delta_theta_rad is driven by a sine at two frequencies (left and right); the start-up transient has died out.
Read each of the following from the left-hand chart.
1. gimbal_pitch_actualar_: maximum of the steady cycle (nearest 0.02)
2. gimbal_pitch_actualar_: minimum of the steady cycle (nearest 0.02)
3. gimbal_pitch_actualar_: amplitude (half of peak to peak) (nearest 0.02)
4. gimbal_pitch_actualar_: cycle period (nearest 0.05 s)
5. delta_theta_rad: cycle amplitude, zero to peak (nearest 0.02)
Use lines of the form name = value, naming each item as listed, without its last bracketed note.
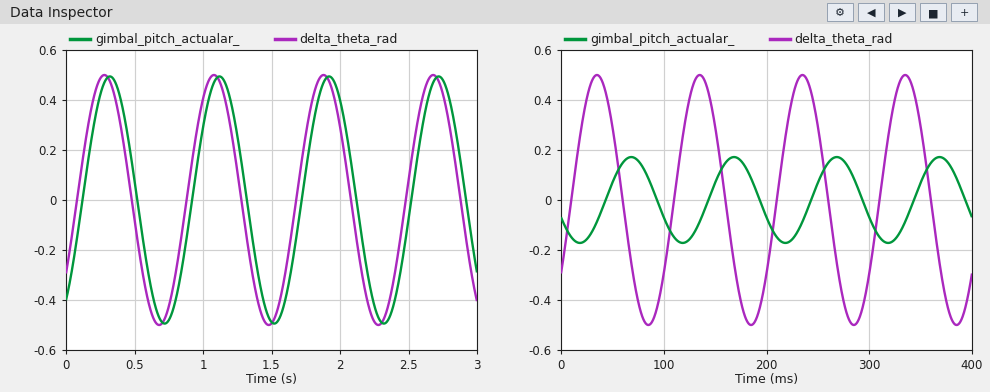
gimbal_pitch_actualar_: maximum of the steady cycle = 0.50
gimbal_pitch_actualar_: minimum of the steady cycle = -0.50
gimbal_pitch_actualar_: amplitude (half of peak to peak) = 0.50
gimbal_pitch_actualar_: cycle period = 0.80 s
delta_theta_rad: cycle amplitude, zero to peak = 0.50
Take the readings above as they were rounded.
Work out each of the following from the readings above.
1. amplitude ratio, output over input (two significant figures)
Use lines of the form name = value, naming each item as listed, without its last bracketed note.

amplitude ratio, output over input = 1.0
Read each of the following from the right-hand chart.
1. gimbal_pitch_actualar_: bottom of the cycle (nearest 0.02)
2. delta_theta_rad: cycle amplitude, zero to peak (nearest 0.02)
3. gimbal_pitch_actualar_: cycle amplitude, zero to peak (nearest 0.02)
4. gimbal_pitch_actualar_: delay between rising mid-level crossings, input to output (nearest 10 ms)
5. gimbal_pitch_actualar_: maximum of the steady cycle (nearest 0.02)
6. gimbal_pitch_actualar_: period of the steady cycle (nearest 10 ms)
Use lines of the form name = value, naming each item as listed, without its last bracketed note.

gimbal_pitch_actualar_: bottom of the cycle = -0.18
delta_theta_rad: cycle amplitude, zero to peak = 0.50
gimbal_pitch_actualar_: cycle amplitude, zero to peak = 0.18
gimbal_pitch_actualar_: delay between rising mid-level crossings, input to output = 30 ms
gimbal_pitch_actualar_: maximum of the steady cycle = 0.18
gimbal_pitch_actualar_: period of the steady cycle = 100 ms
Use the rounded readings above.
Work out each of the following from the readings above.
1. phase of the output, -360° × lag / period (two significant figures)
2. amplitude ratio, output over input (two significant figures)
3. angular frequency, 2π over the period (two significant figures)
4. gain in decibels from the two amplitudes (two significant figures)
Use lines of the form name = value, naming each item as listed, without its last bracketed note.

phase of the output, -360° × lag / period = -110°
amplitude ratio, output over input = 0.36
angular frequency, 2π over the period = 0.063 rad/ms
gain in decibels from the two amplitudes = -8.9 dB
